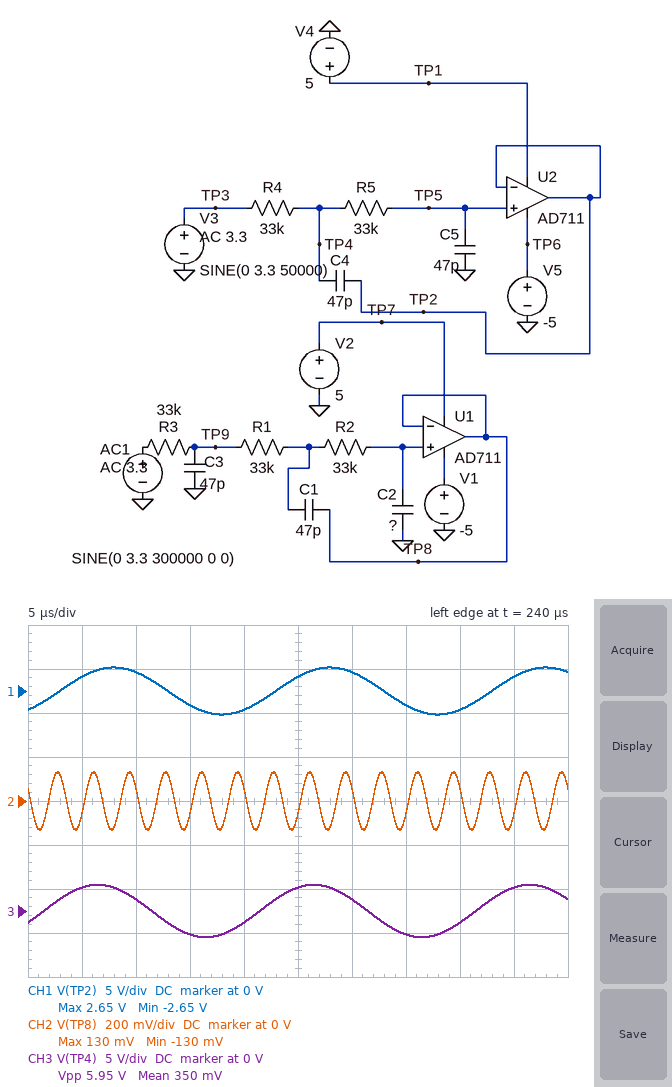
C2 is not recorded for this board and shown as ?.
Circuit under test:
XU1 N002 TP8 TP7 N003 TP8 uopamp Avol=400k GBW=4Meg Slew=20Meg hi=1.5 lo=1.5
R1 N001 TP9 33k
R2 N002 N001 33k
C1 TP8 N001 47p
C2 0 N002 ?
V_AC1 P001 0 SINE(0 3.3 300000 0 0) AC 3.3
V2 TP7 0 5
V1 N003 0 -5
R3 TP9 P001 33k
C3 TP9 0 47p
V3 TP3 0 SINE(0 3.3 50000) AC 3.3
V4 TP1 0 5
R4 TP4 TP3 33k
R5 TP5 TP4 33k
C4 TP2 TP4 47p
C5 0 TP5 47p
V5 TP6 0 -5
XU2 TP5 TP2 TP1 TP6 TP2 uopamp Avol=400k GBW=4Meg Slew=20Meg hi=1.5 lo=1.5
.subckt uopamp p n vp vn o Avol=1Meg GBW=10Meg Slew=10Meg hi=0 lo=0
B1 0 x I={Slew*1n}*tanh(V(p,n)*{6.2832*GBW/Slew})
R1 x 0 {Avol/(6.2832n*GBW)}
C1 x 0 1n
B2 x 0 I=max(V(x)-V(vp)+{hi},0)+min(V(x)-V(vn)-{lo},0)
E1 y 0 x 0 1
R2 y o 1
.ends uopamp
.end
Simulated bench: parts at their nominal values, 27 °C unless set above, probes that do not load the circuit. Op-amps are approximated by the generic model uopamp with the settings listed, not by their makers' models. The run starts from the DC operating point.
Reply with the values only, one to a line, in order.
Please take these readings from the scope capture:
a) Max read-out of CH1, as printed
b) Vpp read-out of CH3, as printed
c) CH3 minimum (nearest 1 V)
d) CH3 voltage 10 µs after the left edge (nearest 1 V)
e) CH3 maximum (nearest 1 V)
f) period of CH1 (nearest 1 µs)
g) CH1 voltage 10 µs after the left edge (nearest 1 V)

2.65 V
5.95 V
-3 V
1 V
3 V
20 µs
2 V
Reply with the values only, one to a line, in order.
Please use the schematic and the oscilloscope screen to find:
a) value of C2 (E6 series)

33 pF
